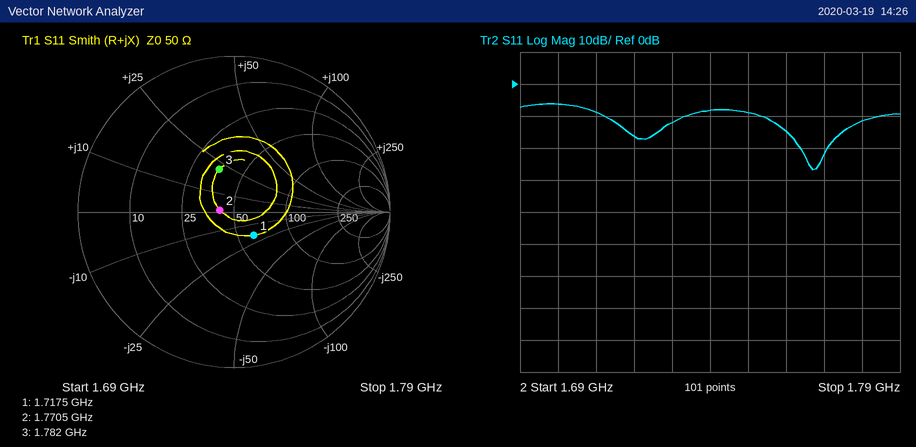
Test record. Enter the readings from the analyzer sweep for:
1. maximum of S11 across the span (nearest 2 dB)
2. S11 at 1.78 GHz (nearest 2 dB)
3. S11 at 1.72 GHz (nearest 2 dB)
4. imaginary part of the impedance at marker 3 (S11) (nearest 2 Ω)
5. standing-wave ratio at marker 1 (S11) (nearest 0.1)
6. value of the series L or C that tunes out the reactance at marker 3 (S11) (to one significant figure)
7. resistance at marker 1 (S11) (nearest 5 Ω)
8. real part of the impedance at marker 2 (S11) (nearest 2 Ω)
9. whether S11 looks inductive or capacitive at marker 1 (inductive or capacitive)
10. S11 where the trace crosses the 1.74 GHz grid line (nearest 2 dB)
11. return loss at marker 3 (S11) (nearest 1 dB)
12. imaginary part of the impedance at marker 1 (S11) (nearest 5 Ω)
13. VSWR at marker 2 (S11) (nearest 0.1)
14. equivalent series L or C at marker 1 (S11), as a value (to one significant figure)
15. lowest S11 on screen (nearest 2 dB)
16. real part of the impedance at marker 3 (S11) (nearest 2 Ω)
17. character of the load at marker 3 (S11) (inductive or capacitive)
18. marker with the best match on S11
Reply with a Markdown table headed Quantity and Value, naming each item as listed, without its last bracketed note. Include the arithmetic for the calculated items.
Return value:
| Quantity | Value |
|---|---|
| maximum of S11 across the span | -6 dB |
| S11 at 1.78 GHz | -12 dB |
| S11 at 1.72 GHz | -16 dB |
| imaginary part of the impedance at marker 3 (S11) | +22 Ω |
| standing-wave ratio at marker 1 (S11) | 1.5 |
| value of the series L or C that tunes out the reactance at marker 3 (S11) | C = 1/(2π × 1.782 GHz × 22 Ω) ≈ 4 pF |
| resistance at marker 1 (S11) | 60 Ω |
| real part of the impedance at marker 2 (S11) | 42 Ω |
| whether S11 looks inductive or capacitive at marker 1 | capacitive |
| S11 where the trace crosses the 1.74 GHz grid line | -8 dB |
| return loss at marker 3 (S11) | 11 dB |
| imaginary part of the impedance at marker 1 (S11) | -20 Ω |
| VSWR at marker 2 (S11) | 1.2 |
| equivalent series L or C at marker 1 (S11), as a value | C = 1/(2π × 1.7175 GHz × 20 Ω) ≈ 5 pF |
| lowest S11 on screen | -26 dB |
| real part of the impedance at marker 3 (S11) | 36 Ω |
| character of the load at marker 3 (S11) | inductive |
| marker with the best match on S11 | marker 2 |
